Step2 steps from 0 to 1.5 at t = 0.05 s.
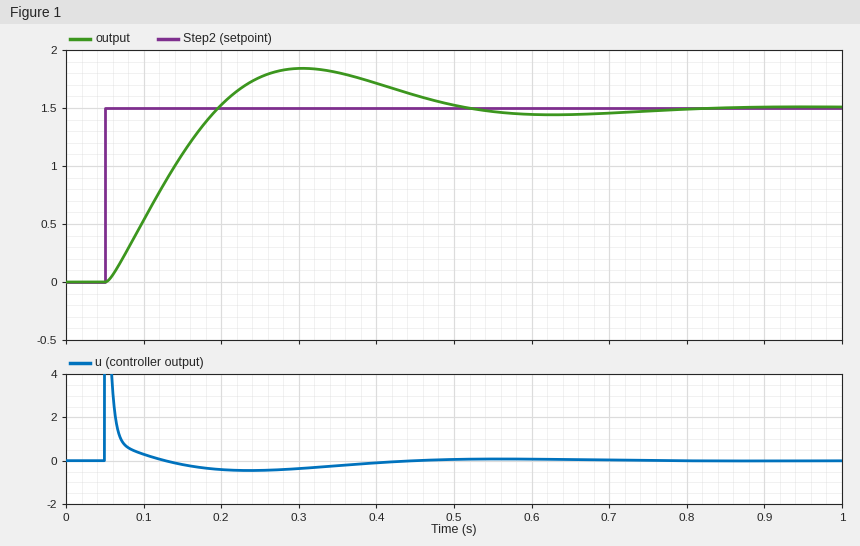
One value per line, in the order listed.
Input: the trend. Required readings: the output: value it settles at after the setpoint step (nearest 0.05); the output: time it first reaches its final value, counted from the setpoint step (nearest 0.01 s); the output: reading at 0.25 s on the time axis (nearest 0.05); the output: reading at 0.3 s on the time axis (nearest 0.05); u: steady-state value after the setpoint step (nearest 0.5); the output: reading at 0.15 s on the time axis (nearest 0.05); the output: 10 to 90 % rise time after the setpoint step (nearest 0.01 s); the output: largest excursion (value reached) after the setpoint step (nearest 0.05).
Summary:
1.50
0.15 s
1.75
1.85
0.0
1.10
0.11 s
1.85
